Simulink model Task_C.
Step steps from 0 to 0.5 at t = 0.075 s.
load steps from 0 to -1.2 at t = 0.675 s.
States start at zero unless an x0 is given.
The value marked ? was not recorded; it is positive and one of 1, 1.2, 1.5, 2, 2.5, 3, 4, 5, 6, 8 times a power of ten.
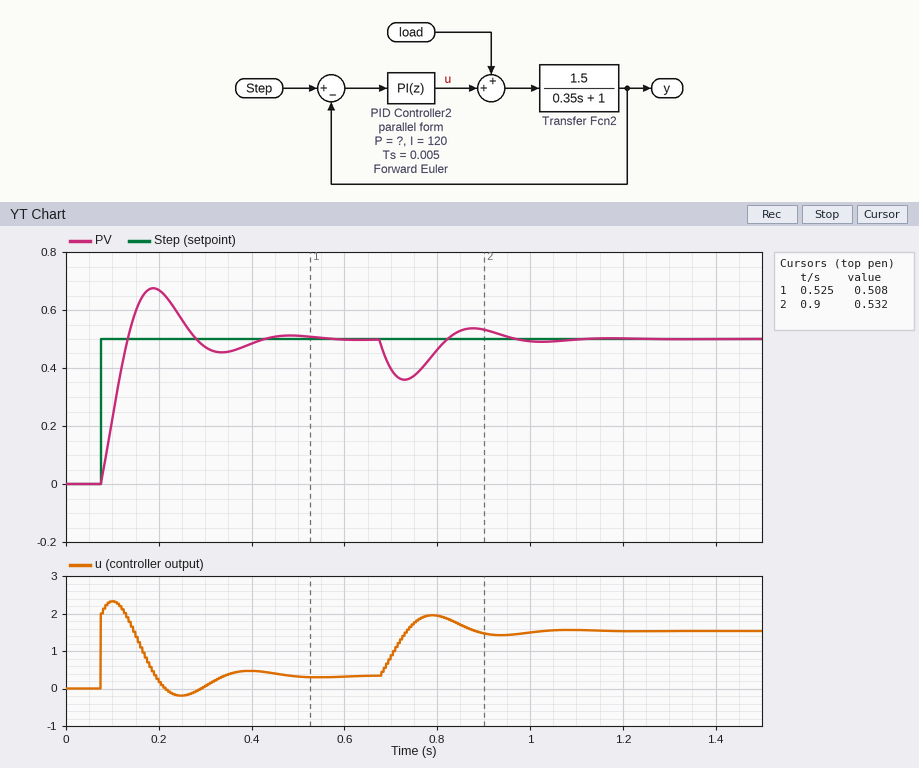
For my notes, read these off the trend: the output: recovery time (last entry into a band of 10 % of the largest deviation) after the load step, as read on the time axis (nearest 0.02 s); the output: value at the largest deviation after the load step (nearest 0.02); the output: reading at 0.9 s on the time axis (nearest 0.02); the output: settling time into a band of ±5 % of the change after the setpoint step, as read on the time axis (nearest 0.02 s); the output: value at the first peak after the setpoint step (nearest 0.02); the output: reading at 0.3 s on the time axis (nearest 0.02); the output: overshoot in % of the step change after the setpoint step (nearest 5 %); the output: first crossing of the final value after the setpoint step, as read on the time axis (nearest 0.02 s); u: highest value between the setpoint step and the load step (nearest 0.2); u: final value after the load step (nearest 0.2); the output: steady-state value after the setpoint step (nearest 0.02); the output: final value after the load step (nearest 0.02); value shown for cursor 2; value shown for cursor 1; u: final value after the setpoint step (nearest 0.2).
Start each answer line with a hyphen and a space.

- 0.94 s
- 0.36
- 0.54
- 0.38 s
- 0.68
- 0.48
- 35 %
- 0.14 s
- 2.4
- 1.6
- 0.50
- 0.50
- 0.532
- 0.508
- 0.4
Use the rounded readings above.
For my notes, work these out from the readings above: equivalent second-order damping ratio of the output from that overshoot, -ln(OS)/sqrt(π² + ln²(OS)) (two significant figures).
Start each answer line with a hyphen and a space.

- 0.32
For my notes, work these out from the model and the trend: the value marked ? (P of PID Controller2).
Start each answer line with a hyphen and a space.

- 4
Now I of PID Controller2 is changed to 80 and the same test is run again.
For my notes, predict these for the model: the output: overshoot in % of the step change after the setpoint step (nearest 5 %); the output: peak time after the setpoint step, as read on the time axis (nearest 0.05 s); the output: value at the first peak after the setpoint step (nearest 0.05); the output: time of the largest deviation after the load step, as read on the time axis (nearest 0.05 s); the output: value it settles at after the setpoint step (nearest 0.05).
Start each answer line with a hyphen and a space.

- 25 %
- 0.20 s
- 0.65
- 0.75 s
- 0.50
